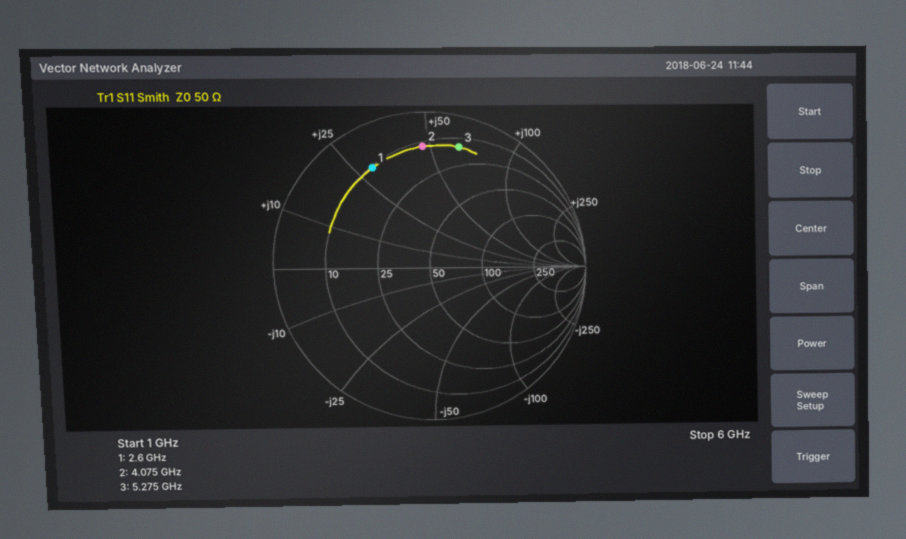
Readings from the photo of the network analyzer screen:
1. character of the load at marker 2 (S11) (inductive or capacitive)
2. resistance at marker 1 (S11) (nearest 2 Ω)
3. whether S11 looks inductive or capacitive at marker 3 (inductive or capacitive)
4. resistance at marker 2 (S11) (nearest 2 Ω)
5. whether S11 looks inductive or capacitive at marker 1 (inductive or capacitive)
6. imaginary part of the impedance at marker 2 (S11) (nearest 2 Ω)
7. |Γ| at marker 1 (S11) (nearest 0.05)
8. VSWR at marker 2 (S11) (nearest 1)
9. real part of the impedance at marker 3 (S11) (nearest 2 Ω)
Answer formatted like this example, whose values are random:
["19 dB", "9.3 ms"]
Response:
["inductive", "10 Ω", "inductive", "12 Ω", "inductive", "+48 Ω", "0.75", "8", "14 Ω"]
